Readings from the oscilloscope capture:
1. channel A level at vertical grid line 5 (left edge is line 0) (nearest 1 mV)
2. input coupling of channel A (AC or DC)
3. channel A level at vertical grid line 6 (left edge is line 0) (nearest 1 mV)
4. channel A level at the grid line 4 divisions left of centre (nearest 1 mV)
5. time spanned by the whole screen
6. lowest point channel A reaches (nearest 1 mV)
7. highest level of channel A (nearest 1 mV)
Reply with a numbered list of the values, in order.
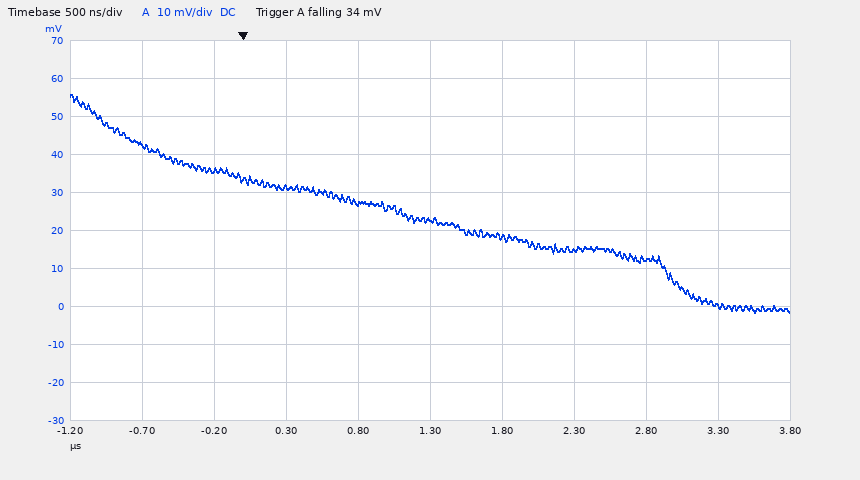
1. 23 mV
2. DC
3. 18 mV
4. 42 mV
5. 5 µs
6. -2 mV
7. 56 mV
